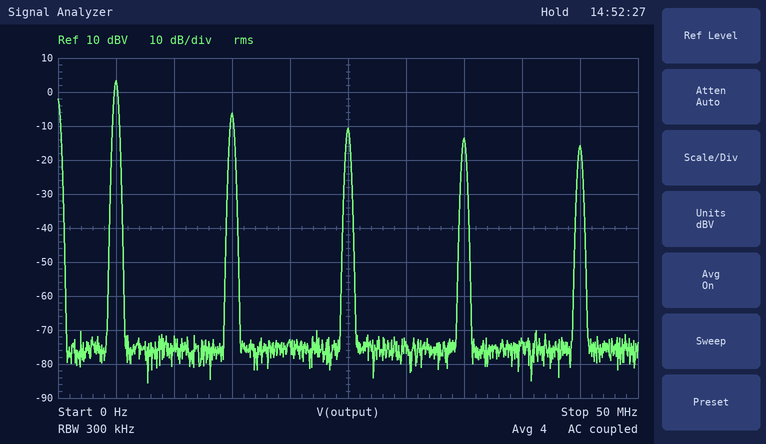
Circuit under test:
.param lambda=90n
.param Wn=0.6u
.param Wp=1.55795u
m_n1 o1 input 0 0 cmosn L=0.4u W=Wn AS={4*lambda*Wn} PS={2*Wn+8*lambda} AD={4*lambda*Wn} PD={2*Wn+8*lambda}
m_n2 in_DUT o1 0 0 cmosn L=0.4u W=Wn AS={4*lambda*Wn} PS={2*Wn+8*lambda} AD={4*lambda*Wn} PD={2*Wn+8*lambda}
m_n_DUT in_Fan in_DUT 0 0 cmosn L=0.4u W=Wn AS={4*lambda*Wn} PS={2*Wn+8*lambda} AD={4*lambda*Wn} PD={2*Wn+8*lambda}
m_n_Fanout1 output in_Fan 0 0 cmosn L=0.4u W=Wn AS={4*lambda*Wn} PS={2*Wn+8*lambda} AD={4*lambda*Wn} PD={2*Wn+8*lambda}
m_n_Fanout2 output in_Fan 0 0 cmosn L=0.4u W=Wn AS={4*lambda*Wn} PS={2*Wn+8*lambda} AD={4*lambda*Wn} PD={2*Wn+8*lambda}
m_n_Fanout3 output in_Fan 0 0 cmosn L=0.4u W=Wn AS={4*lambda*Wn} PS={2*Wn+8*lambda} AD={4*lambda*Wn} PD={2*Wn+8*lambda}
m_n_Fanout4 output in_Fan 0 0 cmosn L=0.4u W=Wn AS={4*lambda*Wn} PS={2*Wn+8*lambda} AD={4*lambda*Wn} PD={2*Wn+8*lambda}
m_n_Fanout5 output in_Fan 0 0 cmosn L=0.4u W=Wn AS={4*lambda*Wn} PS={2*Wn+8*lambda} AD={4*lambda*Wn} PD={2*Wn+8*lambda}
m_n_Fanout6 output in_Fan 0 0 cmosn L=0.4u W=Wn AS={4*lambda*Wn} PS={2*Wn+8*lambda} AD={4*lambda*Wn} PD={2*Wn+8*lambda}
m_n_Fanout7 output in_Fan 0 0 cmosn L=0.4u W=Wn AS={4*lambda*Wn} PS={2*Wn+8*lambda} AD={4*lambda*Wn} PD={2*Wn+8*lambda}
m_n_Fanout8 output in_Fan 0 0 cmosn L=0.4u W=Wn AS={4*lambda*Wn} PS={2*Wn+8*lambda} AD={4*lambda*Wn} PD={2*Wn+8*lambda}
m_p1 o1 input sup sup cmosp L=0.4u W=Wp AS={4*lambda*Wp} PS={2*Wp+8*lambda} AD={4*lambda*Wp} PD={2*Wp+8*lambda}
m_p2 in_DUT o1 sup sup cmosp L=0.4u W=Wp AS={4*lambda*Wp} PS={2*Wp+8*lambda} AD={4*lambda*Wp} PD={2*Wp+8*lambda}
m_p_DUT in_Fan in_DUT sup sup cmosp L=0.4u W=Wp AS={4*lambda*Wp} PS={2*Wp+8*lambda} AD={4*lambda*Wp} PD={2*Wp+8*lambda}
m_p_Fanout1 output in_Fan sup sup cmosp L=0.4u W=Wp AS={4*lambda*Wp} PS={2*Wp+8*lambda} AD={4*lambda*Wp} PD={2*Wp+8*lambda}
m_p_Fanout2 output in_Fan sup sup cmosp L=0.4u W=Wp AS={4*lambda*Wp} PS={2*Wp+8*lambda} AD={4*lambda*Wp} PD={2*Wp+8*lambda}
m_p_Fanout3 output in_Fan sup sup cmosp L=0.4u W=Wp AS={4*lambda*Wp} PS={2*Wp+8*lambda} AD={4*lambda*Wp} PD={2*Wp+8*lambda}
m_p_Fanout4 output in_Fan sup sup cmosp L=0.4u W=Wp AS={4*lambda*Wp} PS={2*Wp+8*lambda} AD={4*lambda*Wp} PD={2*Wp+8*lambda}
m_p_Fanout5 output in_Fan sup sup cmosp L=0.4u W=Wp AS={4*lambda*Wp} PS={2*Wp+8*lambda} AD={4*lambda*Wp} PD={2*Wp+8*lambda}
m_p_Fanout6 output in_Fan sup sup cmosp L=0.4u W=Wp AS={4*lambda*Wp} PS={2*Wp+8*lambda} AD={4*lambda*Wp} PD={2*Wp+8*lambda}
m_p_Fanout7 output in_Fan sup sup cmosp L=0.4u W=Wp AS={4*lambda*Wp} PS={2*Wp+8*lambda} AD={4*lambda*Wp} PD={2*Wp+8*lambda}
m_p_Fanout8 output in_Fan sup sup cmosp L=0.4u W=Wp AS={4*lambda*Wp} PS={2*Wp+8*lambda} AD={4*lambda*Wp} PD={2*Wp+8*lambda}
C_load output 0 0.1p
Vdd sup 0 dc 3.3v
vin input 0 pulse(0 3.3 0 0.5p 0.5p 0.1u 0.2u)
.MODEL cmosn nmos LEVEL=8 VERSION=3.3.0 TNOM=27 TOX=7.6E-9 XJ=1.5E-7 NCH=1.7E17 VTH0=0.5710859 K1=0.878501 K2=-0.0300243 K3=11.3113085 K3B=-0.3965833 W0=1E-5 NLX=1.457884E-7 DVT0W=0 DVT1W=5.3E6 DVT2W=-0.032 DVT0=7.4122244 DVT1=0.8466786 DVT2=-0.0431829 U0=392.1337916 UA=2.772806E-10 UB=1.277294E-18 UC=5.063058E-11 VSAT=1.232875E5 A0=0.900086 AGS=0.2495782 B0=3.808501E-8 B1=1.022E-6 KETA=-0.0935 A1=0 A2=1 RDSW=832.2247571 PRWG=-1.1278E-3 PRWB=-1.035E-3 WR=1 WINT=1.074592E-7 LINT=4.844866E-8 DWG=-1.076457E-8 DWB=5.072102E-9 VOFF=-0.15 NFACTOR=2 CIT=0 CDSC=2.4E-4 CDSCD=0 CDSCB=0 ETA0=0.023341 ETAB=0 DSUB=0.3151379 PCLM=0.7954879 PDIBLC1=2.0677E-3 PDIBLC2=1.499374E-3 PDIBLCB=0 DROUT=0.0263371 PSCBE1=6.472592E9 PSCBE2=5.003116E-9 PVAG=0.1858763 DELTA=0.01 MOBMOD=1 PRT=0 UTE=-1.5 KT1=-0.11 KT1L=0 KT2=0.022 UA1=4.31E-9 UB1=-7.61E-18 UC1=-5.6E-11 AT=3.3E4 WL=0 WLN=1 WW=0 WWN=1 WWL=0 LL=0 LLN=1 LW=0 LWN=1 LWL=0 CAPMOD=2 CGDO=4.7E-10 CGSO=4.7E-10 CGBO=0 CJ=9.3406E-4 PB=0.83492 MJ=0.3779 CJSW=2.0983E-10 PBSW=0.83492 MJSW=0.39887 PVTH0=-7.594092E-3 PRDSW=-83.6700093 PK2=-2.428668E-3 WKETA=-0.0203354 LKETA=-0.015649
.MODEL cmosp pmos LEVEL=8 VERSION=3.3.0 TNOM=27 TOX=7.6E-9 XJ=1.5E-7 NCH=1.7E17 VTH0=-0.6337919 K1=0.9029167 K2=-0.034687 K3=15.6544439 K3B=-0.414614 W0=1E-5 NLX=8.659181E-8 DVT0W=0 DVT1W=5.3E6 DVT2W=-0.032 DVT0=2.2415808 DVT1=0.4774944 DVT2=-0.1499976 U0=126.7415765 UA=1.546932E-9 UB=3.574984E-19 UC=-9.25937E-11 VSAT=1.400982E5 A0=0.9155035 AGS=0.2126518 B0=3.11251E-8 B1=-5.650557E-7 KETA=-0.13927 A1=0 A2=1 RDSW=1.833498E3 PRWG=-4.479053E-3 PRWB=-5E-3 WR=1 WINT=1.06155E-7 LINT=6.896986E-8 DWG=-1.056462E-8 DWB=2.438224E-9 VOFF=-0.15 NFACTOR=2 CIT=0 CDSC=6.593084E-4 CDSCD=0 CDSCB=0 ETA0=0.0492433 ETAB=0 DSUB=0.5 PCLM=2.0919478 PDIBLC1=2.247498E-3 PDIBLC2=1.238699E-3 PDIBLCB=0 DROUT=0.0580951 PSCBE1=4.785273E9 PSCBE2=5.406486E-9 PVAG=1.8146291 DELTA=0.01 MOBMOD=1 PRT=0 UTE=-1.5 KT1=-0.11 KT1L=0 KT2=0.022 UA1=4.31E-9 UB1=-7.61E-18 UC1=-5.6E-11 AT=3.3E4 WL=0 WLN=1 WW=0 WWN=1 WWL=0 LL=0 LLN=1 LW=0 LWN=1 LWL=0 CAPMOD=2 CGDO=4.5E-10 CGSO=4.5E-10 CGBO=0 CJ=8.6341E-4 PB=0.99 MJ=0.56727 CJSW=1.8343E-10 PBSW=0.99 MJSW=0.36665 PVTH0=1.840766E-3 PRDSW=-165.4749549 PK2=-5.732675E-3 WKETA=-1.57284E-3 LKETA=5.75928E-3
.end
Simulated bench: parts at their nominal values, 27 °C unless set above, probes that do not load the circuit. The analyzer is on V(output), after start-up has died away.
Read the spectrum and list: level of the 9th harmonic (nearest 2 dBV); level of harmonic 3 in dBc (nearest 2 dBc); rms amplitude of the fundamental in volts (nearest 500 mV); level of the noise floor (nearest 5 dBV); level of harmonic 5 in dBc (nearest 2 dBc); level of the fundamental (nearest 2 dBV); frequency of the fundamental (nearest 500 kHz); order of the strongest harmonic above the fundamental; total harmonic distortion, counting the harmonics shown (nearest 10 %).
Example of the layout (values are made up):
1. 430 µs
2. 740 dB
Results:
1. -16 dBV
2. -10 dBc
3. 1.5 V
4. -75 dBV
5. -14 dBc
6. 4 dBV
7. 5.0 MHz
8. 3
9. 40 %
